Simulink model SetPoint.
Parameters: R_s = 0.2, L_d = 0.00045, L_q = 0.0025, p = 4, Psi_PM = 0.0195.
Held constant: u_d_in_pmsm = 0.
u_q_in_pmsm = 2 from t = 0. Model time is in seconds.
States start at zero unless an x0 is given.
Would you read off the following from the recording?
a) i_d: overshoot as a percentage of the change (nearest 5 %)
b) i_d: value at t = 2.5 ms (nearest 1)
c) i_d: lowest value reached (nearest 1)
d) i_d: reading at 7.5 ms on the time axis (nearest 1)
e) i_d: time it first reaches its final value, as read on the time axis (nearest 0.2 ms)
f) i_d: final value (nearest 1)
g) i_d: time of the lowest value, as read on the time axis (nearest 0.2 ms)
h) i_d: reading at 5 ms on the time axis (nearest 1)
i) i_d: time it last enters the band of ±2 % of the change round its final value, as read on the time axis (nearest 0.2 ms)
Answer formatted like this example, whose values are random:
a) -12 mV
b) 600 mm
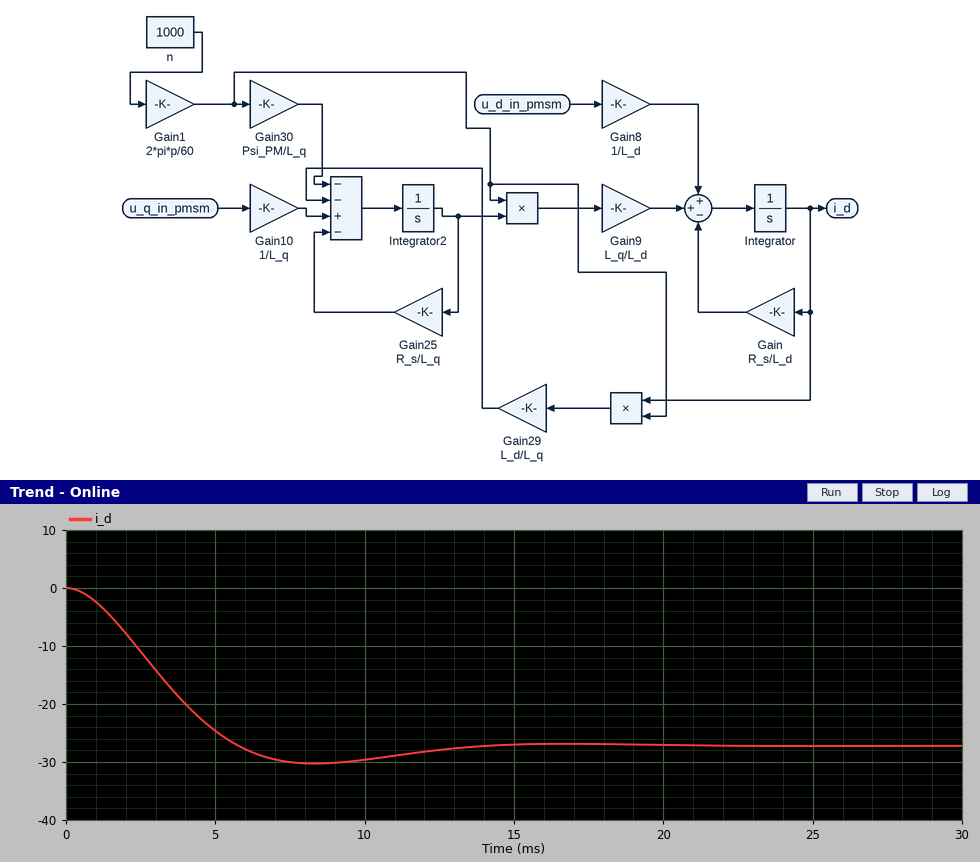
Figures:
a) 10 %
b) -11
c) -30
d) -30
e) 5.8 ms
f) -27
g) 8.4 ms
h) -25
i) 12.8 ms
